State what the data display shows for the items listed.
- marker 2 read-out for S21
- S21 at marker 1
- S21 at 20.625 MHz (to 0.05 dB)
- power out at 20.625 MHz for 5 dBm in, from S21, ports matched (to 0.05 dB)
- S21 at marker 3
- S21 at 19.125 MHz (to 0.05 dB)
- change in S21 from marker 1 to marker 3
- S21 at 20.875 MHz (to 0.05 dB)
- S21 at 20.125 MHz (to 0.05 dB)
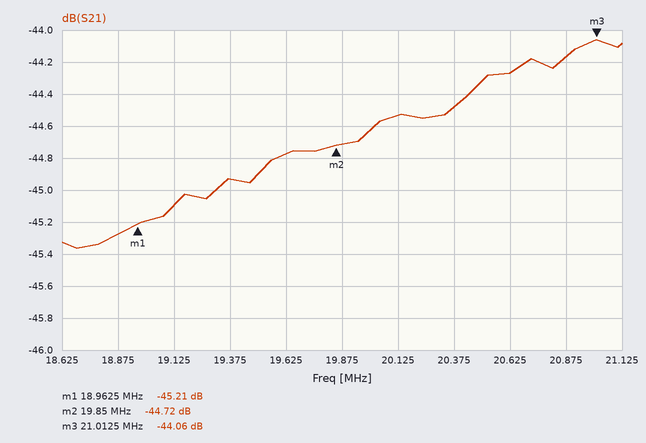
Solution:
-44.72 dB
-45.21 dB
-44.25 dB
-39.25 dBm
-44.06 dB
-45.10 dB
1.15 dB
-44.15 dB
-44.55 dB
